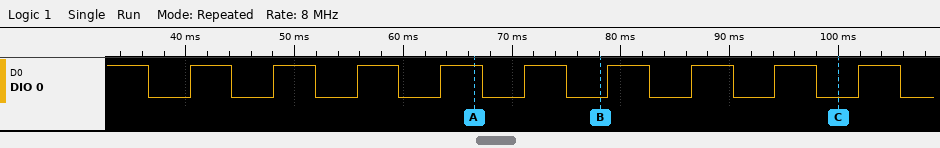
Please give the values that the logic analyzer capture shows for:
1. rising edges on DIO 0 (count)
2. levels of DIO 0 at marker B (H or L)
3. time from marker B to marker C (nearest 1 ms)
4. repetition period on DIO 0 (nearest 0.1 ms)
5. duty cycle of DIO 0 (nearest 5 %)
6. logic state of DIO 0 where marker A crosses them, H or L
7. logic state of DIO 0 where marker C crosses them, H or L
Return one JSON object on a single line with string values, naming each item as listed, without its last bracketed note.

{"rising edges on DIO 0": "9", "levels of DIO 0 at marker B": "DIO 0=L", "time from marker B to marker C": "22 ms", "repetition period on DIO 0": "7.7 ms", "duty cycle of DIO 0": "50 %", "logic state of DIO 0 where marker A crosses them, H or L": "DIO 0=H", "logic state of DIO 0 where marker C crosses them, H or L": "DIO 0=L"}
